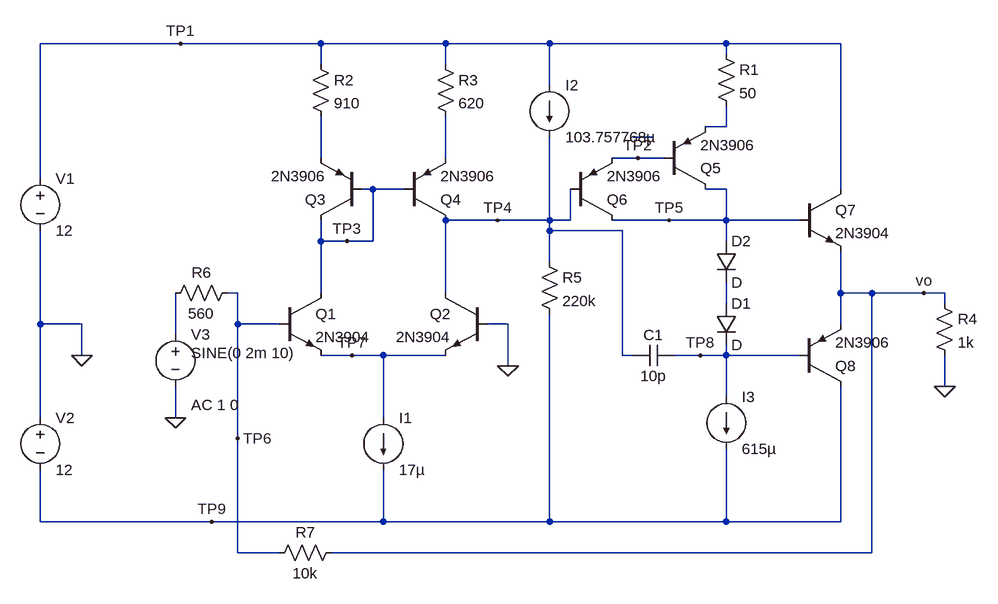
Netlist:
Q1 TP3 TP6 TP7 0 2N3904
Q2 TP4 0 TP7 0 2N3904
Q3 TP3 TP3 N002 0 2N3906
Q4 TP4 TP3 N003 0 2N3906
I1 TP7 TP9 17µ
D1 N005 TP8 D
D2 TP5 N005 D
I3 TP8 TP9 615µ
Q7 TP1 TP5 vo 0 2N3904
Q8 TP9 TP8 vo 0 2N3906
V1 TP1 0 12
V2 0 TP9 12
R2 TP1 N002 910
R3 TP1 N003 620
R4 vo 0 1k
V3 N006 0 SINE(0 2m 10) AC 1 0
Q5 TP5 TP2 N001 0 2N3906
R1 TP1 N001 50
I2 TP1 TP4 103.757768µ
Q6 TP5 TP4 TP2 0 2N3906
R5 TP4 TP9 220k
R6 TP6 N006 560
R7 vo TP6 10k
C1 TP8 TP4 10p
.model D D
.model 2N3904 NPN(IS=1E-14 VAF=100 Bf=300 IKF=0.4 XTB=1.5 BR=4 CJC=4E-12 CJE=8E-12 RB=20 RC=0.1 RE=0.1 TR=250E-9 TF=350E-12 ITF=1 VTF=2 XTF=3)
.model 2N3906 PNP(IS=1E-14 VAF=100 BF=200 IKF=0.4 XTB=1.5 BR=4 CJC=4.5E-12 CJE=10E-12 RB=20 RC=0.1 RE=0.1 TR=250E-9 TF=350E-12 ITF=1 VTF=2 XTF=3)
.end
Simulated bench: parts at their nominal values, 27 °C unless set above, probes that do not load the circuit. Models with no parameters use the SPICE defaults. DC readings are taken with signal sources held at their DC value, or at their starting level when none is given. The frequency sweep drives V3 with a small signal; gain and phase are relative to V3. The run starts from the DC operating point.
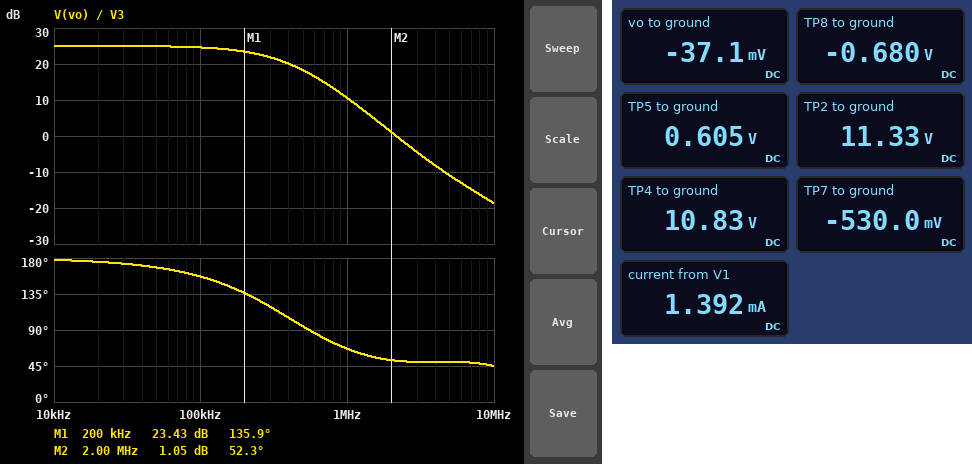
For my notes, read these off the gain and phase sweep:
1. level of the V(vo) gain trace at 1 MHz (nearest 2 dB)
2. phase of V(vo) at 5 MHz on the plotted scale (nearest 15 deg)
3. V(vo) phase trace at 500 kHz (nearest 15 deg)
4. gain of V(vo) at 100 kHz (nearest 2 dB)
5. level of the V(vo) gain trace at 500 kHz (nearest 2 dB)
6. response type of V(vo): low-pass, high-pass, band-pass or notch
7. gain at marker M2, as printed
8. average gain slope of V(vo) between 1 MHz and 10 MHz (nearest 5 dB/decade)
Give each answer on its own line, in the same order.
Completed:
10 dB
45 deg
90 deg
24 dB
18 dB
low-pass
1.05 dB
-30 dB/decade
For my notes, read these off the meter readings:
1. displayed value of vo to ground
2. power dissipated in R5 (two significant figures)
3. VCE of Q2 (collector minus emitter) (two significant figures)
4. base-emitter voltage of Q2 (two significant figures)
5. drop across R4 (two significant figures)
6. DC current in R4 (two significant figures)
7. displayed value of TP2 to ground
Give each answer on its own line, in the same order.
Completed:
-37.1 mV
2.4 mW
11 V
530 mV
37 mV
37 µA
11.33 V
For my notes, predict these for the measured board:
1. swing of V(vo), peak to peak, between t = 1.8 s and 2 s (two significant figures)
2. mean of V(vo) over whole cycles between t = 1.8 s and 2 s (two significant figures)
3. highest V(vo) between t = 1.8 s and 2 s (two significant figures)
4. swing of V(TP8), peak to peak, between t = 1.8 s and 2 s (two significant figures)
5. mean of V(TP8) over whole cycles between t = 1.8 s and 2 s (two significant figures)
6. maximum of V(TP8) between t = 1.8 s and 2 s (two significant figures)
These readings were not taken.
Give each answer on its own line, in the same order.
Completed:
71 mV
-37 mV
-1.4 mV
73 mV
-680 mV
-640 mV
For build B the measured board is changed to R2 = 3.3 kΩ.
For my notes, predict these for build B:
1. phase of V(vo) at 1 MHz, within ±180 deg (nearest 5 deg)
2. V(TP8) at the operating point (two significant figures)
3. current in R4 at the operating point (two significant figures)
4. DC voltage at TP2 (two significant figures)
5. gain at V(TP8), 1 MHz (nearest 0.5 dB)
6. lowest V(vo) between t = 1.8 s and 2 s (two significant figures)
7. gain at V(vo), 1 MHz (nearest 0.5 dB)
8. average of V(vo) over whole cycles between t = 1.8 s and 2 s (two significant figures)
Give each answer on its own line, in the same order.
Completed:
55 deg
-910 mV
260 µA
11 V
13.0 dB
-300 mV
12.5 dB
-260 mV
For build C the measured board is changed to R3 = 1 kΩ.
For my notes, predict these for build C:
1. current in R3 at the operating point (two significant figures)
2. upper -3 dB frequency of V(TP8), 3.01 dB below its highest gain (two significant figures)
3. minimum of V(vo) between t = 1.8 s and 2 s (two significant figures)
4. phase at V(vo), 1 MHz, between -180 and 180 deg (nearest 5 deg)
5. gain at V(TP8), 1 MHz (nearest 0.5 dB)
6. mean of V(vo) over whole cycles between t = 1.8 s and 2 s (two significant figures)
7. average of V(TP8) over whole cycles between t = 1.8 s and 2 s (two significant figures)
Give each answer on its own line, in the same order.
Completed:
8.4 µA
260 kHz
-25 mV
70 deg
10.0 dB
11 mV
-630 mV
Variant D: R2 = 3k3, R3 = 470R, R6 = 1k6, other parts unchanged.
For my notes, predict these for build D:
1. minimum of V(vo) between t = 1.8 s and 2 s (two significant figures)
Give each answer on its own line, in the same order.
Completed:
-120 mV
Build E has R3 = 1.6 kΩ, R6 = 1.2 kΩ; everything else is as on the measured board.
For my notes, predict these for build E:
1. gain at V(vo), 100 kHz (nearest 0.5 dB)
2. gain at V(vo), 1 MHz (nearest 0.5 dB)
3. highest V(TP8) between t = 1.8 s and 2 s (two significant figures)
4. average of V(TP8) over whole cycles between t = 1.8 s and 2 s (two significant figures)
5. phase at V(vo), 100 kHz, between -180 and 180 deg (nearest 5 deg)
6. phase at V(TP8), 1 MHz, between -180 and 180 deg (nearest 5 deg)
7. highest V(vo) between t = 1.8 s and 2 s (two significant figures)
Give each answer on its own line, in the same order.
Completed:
18.5 dB
9.0 dB
-590 mV
-600 mV
165 deg
75 deg
55 mV
